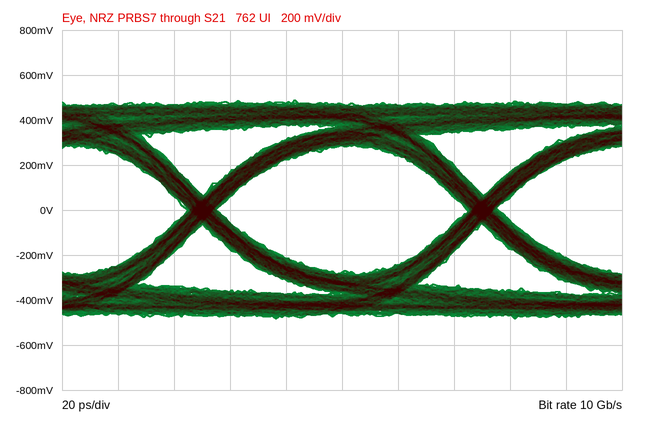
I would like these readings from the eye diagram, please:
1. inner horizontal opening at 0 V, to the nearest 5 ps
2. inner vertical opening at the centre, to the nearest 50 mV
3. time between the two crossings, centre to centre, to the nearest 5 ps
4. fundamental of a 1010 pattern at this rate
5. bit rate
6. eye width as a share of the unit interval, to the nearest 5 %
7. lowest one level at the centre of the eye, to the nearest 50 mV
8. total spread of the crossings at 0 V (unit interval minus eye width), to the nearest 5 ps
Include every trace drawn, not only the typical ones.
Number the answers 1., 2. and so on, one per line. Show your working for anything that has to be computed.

1. 90 ps
2. 550 mV
3. 100 ps
4. 5 GHz
5. 10 Gb/s
6. 90 ps / 100 ps ≈ 90 %
7. 300 mV
8. 10 ps
